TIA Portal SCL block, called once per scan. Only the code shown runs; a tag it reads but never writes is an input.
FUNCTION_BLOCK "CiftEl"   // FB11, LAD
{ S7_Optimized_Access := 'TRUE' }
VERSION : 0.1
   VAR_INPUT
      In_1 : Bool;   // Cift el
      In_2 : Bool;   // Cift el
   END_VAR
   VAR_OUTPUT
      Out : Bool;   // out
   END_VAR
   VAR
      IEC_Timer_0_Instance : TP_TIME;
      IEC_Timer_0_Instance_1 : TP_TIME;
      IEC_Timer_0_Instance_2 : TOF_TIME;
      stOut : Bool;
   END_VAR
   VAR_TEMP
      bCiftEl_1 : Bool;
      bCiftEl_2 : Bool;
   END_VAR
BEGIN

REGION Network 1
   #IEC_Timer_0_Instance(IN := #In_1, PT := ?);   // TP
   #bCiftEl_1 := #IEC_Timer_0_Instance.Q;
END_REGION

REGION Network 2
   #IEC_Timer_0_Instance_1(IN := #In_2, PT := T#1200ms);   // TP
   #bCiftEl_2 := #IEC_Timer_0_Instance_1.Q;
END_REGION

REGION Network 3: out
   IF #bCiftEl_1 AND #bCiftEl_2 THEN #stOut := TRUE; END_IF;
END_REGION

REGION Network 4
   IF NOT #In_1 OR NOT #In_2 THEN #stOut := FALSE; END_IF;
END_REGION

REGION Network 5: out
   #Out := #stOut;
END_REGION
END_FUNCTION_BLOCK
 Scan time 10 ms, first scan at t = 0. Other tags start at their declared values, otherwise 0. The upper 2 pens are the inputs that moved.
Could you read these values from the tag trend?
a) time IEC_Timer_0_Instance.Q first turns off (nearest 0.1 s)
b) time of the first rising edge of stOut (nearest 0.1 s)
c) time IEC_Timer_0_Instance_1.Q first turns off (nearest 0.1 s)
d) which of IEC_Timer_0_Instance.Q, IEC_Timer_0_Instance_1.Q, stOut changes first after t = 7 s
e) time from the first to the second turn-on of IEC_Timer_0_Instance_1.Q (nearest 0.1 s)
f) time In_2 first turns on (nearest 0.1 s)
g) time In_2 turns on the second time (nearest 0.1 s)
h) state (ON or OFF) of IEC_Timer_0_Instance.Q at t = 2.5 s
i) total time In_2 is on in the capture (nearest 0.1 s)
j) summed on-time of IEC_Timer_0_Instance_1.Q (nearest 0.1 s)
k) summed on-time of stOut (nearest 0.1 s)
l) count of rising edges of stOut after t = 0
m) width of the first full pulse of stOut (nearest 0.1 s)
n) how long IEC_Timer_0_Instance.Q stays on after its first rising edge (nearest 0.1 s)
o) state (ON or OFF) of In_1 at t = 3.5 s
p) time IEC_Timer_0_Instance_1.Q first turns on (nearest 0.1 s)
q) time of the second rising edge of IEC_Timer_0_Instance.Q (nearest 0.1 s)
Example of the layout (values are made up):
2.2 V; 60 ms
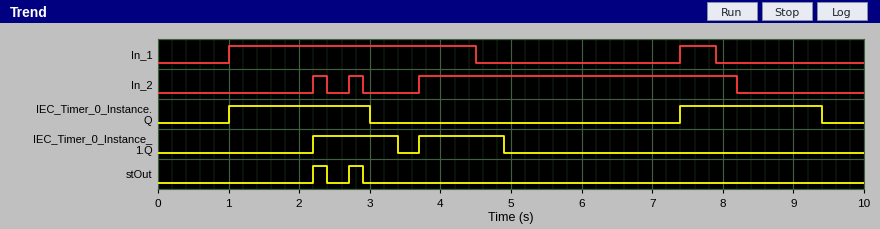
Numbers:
3.0 s; 2.2 s; 3.4 s; IEC_Timer_0_Instance.Q; 1.5 s; 2.2 s; 2.7 s; ON; 4.9 s; 2.4 s; 0.4 s; 2; 0.2 s; 2.0 s; ON; 2.2 s; 7.4 s
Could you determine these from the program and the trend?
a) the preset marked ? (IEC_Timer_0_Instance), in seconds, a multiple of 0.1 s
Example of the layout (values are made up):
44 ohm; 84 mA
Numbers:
2.0 s
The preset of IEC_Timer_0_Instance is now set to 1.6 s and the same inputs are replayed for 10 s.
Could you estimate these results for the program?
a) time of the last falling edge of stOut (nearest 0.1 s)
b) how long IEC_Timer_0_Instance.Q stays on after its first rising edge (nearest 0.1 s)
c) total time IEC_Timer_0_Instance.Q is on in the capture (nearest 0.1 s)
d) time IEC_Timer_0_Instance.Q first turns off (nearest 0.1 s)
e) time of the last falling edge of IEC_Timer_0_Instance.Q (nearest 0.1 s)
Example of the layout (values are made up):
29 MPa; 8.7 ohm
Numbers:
2.4 s; 1.6 s; 3.2 s; 2.6 s; 9.0 s
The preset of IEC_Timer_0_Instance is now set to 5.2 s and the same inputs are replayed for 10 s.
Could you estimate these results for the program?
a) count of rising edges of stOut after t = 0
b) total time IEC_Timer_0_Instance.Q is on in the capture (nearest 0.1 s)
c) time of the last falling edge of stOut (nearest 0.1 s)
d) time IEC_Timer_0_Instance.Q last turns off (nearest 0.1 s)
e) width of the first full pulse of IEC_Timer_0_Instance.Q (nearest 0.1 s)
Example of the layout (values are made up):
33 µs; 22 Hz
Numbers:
3; 7.8 s; 4.5 s; 6.2 s; 5.2 s
